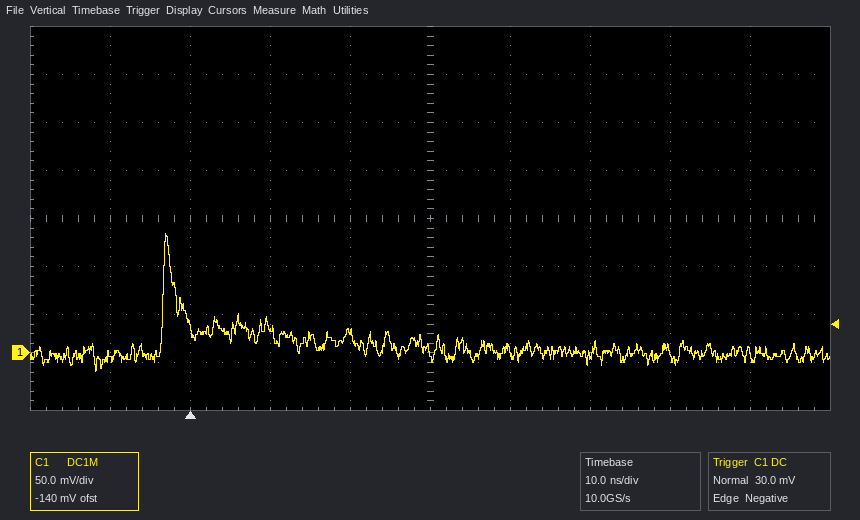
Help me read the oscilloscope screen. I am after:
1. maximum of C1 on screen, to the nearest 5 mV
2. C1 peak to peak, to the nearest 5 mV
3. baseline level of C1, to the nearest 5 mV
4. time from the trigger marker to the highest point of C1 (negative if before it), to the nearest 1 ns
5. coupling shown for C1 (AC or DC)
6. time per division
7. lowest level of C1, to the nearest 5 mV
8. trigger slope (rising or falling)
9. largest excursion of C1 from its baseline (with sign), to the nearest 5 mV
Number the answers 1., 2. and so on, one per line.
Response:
1. 125 mV
2. 145 mV
3. 0 mV
4. -3 ns
5. DC
6. 10 ns
7. -20 mV
8. falling
9. +125 mV
